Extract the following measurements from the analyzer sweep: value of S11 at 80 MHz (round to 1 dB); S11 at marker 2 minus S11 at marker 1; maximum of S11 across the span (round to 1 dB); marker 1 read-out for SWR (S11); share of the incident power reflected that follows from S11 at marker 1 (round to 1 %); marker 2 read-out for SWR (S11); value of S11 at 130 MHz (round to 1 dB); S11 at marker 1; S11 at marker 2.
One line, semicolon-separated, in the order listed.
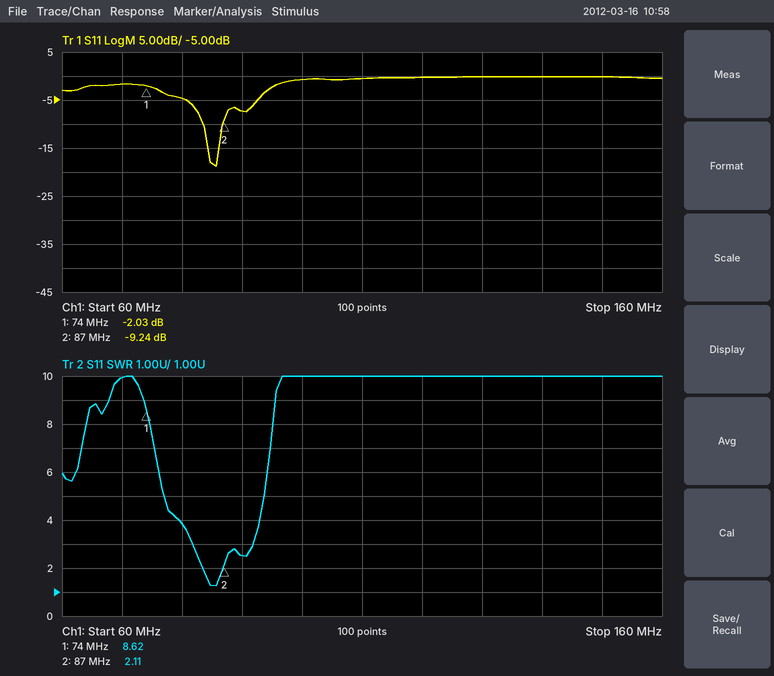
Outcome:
-5 dB; -7.21 dB; 0 dB; 8.62; 63 %; 2.11; 0 dB; -2.03 dB; -9.24 dB
